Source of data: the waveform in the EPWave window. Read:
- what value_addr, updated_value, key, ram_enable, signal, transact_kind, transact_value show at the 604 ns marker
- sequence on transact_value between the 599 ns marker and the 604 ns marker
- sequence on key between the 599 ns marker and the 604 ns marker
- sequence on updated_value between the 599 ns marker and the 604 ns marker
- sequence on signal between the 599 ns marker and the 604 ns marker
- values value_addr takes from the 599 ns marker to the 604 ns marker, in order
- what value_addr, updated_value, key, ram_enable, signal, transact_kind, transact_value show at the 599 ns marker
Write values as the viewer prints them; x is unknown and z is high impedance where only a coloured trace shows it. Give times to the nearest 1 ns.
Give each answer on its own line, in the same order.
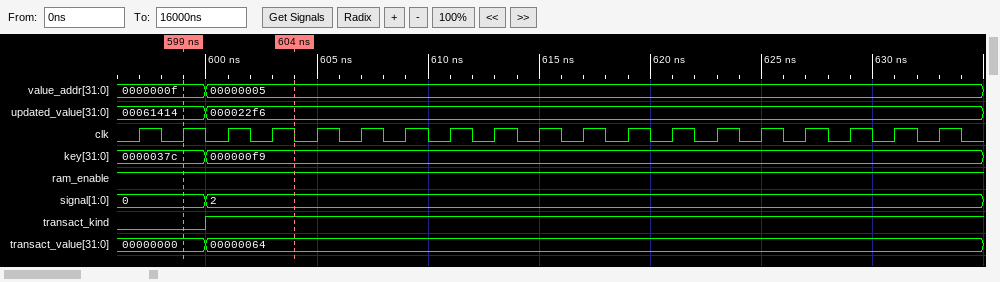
value_addr=00000005, updated_value=000022f6, key=000000f9, ram_enable=1, signal=2, transact_kind=1, transact_value=00000064
00000000, 00000064
0000037c, 000000f9
00061414, 000022f6
0, 2
0000000f, 00000005
value_addr=0000000f, updated_value=00061414, key=0000037c, ram_enable=1, signal=0, transact_kind=0, transact_value=00000000
